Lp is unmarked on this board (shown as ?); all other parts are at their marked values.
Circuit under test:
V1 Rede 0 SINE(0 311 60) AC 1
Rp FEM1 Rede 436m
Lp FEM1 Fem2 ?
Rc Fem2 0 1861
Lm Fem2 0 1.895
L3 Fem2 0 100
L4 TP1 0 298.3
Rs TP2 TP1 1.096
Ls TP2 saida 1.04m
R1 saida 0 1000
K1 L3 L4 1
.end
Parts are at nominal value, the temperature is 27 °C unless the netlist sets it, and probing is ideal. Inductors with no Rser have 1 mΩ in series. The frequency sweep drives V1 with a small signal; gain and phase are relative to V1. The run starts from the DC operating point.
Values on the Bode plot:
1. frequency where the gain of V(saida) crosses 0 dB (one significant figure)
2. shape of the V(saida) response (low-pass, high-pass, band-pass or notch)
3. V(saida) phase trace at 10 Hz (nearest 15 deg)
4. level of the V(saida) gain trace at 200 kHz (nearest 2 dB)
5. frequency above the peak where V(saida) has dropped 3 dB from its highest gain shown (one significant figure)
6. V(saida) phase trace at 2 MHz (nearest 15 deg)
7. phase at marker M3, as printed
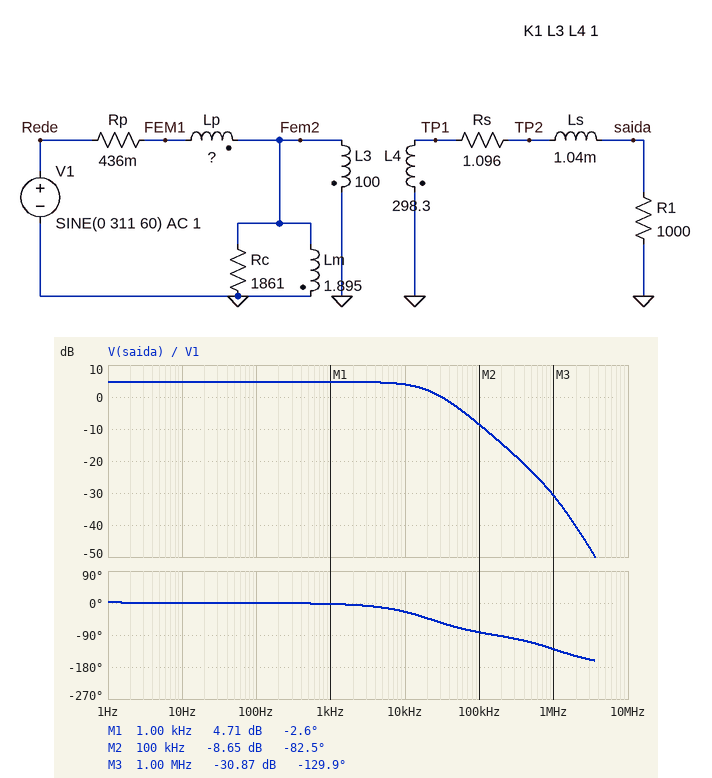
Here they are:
30 kHz
low-pass
0 deg
-14 dB
20 kHz
-150 deg
-129.9 deg
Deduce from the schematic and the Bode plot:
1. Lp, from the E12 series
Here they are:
1.8 mH
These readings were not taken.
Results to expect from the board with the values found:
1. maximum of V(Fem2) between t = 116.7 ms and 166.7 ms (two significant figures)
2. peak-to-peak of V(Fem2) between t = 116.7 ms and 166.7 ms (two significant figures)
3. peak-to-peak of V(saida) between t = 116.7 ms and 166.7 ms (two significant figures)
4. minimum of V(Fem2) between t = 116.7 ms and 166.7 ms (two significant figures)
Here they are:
310 V
620 V
1.1 kV
-310 V
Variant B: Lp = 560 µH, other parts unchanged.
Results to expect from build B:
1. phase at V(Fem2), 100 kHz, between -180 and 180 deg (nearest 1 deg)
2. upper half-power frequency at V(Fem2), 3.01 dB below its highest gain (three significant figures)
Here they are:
-32 deg
63.6 kHz
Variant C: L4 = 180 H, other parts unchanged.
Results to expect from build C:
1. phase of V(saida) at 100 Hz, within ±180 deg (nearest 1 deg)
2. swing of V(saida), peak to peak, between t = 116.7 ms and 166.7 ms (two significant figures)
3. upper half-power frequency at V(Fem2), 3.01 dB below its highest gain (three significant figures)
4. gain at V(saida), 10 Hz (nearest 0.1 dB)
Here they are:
0 deg
830 V
33.0 kHz
2.5 dB
